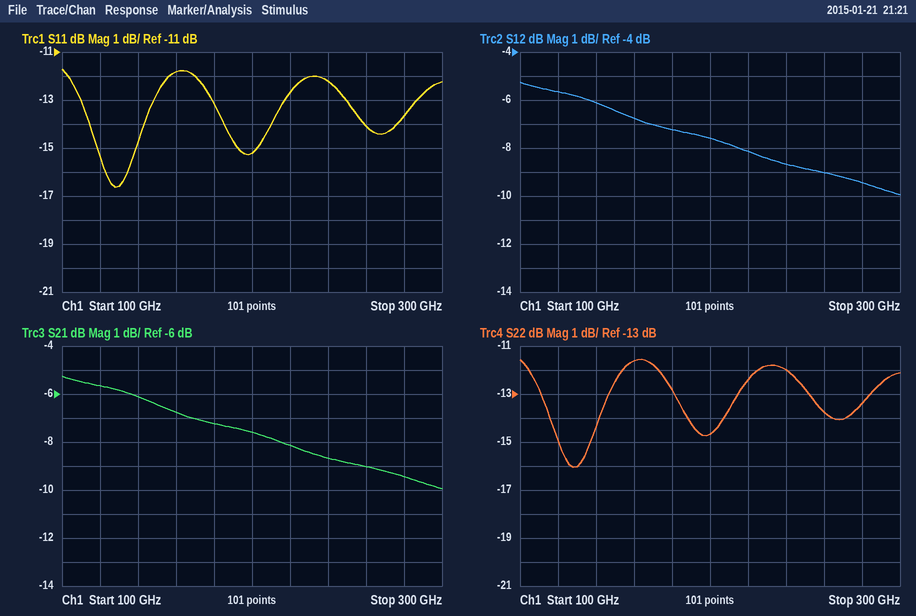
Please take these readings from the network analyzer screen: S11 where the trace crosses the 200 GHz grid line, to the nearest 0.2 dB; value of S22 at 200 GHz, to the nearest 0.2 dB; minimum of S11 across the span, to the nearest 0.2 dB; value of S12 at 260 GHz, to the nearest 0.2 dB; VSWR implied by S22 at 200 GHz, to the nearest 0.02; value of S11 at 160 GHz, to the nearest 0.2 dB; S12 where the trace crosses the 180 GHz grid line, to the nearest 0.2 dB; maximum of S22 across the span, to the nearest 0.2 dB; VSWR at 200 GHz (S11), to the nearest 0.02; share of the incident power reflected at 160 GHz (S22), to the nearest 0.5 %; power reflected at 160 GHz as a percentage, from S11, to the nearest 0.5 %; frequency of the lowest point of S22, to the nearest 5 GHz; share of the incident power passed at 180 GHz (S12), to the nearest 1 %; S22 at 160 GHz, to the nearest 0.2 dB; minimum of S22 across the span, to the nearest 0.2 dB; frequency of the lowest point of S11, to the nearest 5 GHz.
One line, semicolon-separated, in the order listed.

-15.2 dB; -14.6 dB; -16.6 dB; -9.0 dB; 1.46; -11.8 dB; -7.2 dB; -11.6 dB; 1.42; 7.0 %; 6.5 %; 130 GHz; 19 %; -11.6 dB; -16.0 dB; 130 GHz
